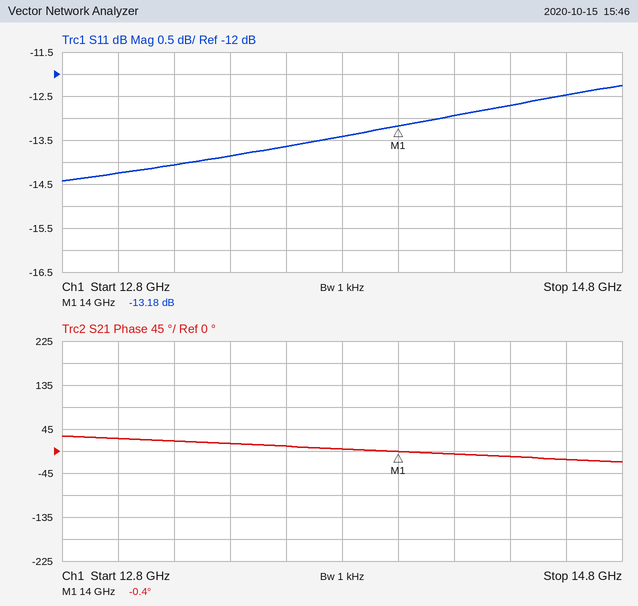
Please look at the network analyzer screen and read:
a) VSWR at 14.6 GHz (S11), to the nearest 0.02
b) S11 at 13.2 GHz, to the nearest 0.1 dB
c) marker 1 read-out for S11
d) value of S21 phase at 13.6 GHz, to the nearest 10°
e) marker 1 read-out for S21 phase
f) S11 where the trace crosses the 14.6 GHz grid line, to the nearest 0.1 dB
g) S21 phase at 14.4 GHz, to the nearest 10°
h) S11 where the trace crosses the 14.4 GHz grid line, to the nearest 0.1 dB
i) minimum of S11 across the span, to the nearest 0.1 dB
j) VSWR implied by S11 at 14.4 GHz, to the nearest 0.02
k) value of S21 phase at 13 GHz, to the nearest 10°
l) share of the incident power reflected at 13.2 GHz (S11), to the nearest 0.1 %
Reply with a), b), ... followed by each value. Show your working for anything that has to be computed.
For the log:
a) |Γ| = 10^(-12.5/20) = 0.2371; VSWR = (1 + 0.2371)/(1 − 0.2371) ≈ 1.62
b) -14.1 dB
c) -13.18 dB
d) 10°
e) -0.4°
f) -12.5 dB
g) -10°
h) -12.7 dB
i) -14.4 dB
j) |Γ| = 10^(-12.7/20) = 0.2317; VSWR = (1 + 0.2317)/(1 − 0.2317) ≈ 1.60
k) 30°
l) 10^(-14.1/10) ≈ 3.9 %
